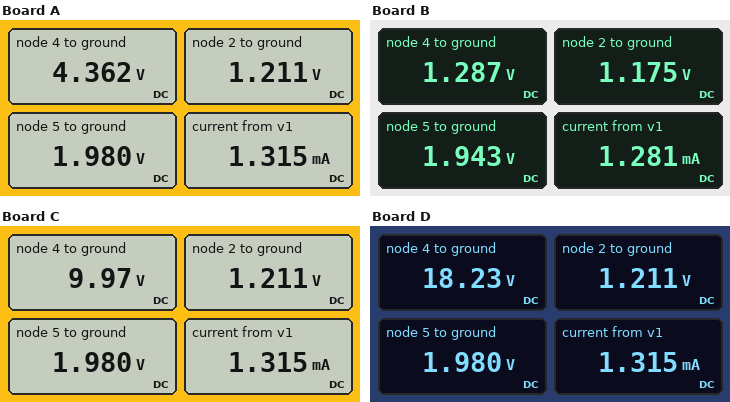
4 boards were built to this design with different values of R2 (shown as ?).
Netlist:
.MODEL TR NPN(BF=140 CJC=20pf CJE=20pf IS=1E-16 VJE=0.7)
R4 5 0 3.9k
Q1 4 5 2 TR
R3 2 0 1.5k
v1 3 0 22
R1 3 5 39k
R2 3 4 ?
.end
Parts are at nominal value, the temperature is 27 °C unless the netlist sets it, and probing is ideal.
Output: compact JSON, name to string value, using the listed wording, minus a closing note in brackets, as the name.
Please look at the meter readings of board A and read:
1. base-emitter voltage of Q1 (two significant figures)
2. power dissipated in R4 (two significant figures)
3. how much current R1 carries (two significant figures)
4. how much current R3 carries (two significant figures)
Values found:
{"base-emitter voltage of Q1": "770 mV", "power dissipated in R4": "1.0 mW", "how much current R1 carries": "510 µA", "how much current R3 carries": "810 µA"}
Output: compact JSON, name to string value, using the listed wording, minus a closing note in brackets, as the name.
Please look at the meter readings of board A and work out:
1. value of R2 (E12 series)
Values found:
{"value of R2": "22 kΩ"}
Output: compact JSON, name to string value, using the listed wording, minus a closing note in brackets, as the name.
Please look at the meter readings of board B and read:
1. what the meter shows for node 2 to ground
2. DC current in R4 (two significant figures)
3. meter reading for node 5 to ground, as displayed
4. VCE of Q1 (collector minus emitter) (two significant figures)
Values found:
{"what the meter shows for node 2 to ground": "1.175 V", "DC current in R4": "500 µA", "meter reading for node 5 to ground, as displayed": "1.943 V", "VCE of Q1 (collector minus emitter)": "110 mV"}
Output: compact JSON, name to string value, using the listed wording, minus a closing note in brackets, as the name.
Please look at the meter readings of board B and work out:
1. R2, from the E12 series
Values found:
{"R2, from the E12 series": "27 kΩ"}
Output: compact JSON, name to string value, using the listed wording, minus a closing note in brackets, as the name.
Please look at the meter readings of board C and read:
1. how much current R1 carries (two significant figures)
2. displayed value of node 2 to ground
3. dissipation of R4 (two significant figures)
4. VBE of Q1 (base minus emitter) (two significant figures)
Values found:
{"how much current R1 carries": "510 µA", "displayed value of node 2 to ground": "1.211 V", "dissipation of R4": "1.0 mW", "VBE of Q1 (base minus emitter)": "770 mV"}
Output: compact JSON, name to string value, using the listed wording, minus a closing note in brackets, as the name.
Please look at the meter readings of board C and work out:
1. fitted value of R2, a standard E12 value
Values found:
{"fitted value of R2, a standard E12 value": "15 kΩ"}
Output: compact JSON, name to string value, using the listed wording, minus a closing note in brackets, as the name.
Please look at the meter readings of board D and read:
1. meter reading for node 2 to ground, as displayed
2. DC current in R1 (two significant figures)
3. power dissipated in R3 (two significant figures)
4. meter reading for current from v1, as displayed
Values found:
{"meter reading for node 2 to ground, as displayed": "1.211 V", "DC current in R1": "510 µA", "power dissipated in R3": "980 µW", "meter reading for current from v1, as displayed": "1.315 mA"}
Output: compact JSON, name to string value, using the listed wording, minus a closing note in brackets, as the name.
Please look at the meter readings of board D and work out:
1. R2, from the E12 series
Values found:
{"R2, from the E12 series": "4.7 kΩ"}
